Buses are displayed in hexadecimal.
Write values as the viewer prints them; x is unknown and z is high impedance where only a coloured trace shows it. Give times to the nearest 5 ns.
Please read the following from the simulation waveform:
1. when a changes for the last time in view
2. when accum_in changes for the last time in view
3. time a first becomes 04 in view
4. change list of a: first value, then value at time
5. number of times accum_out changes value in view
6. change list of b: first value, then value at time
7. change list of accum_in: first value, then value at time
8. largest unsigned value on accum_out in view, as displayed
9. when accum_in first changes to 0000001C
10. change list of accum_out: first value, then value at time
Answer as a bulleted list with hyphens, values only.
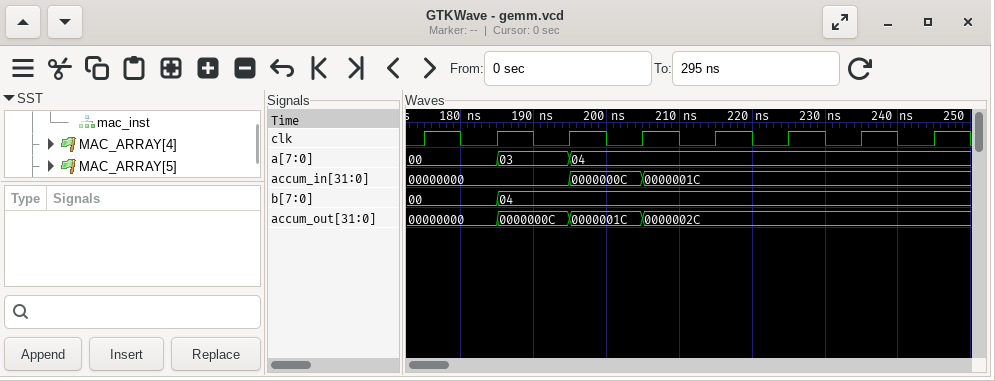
- 195 ns
- 205 ns
- 195 ns
- 00, 03 at 185 ns, 04 at 195 ns
- 3
- 00, 04 at 185 ns
- 00000000, 0000000C at 195 ns, 0000001C at 205 ns
- 0000002C
- 205 ns
- 00000000, 0000000C at 185 ns, 0000001C at 195 ns, 0000002C at 205 ns
